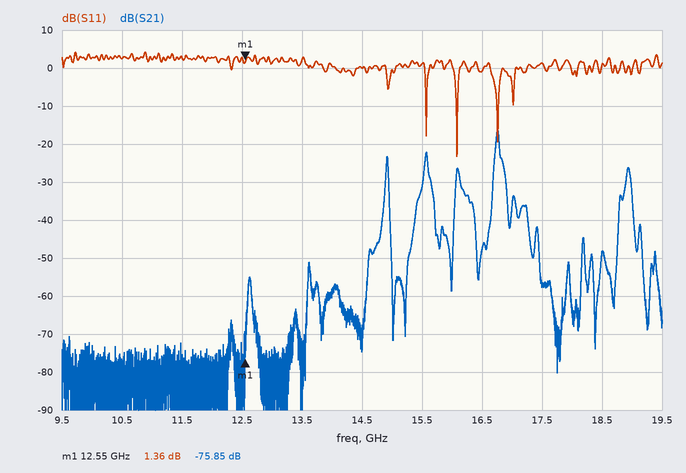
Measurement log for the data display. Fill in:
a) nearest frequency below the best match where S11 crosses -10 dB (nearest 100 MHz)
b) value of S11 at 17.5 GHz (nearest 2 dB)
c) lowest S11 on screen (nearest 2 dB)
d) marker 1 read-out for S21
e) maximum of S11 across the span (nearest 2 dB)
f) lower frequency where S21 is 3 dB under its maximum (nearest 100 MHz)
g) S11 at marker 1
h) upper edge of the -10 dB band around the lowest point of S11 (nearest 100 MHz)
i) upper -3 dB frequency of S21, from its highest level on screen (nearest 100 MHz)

16.1 GHz
2 dB
-24 dB
-75.85 dB
4 dB
16.7 GHz
1.36 dB
16.1 GHz
16.8 GHz
